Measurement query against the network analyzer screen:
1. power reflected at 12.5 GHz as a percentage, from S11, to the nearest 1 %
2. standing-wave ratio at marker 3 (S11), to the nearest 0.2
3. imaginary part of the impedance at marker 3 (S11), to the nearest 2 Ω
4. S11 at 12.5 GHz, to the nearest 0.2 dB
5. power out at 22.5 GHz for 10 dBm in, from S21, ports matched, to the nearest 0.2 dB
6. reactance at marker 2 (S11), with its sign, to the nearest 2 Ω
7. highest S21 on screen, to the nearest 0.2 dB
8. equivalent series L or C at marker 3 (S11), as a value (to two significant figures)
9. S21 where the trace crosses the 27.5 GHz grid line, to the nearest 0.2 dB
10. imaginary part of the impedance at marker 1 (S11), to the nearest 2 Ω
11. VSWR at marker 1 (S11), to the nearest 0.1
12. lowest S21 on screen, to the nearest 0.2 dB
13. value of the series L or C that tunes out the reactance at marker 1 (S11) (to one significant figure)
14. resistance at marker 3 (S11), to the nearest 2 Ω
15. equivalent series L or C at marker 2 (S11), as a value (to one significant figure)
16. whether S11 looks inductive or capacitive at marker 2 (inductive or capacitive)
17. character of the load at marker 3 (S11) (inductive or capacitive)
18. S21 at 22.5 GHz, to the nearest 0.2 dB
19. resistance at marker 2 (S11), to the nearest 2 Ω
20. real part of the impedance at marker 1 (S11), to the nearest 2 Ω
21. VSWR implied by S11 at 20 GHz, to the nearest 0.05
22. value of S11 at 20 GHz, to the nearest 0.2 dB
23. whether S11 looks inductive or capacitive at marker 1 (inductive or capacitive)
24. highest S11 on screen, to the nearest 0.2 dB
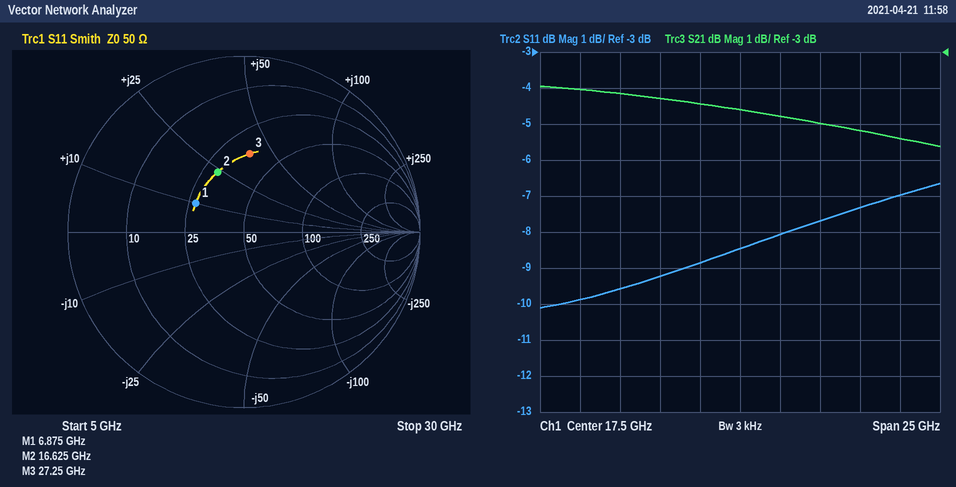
12 %
2.6
+40 Ω
-9.2 dB
5.0 dBm
+24 Ω
-4.0 dB
230 pH
-5.4 dB
+10 Ω
1.9
-5.6 dB
2 pF
36 Ω
200 pH
inductive
inductive
-5.0 dB
30 Ω
28 Ω
2.30
-8.0 dB
inductive
-6.6 dB
